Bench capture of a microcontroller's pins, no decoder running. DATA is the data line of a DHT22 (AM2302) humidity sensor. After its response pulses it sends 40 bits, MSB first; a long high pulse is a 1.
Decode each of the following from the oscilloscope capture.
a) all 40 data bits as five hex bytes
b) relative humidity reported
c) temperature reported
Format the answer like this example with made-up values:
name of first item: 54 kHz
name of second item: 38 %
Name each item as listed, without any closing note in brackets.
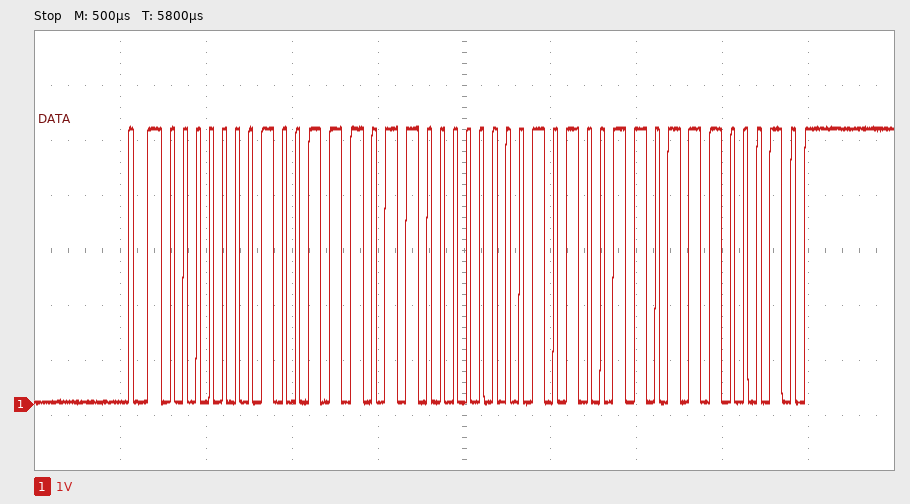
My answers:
all 40 data bits as five hex bytes: 01 3B 00 A6 E2
relative humidity reported: 31.5 %
temperature reported: 16.6 °C
